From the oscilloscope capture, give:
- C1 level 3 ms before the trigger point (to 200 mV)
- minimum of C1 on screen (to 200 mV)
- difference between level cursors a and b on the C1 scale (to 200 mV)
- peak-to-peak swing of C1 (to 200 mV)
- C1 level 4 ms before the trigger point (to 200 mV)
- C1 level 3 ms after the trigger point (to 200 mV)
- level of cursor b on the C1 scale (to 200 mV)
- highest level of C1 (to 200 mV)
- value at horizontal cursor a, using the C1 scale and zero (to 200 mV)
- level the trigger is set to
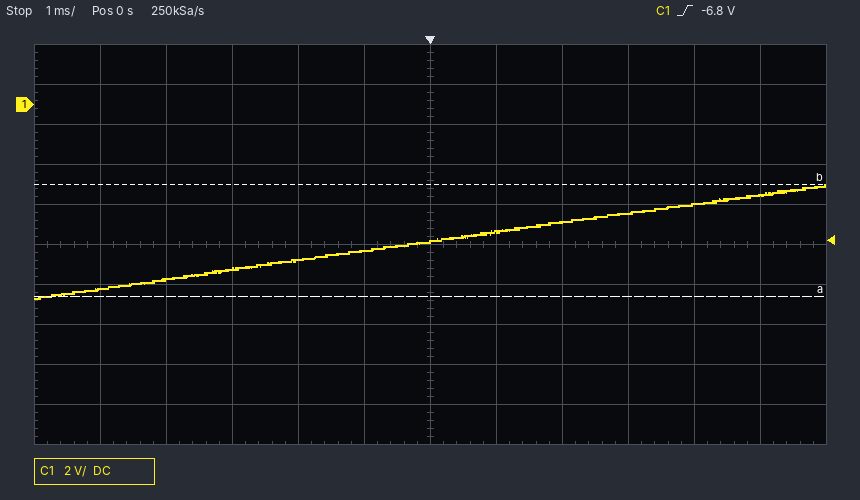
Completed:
-8.2 V
-9.6 V
5.6 V
5.6 V
-8.8 V
-5.4 V
-4.0 V
-4.0 V
-9.6 V
-6.8 V
